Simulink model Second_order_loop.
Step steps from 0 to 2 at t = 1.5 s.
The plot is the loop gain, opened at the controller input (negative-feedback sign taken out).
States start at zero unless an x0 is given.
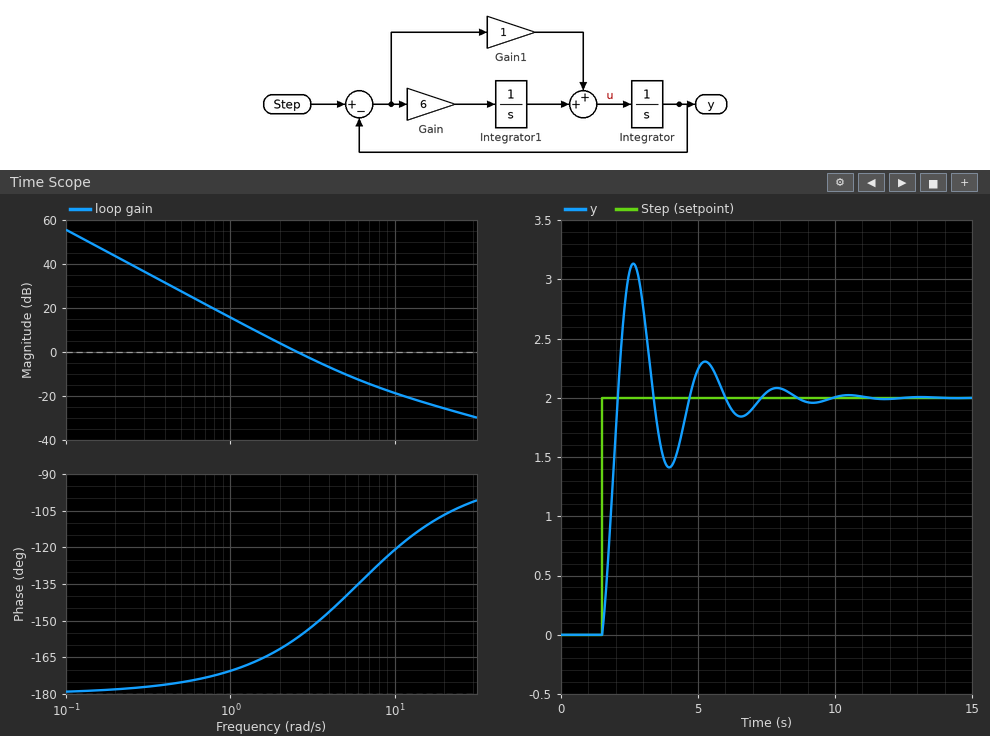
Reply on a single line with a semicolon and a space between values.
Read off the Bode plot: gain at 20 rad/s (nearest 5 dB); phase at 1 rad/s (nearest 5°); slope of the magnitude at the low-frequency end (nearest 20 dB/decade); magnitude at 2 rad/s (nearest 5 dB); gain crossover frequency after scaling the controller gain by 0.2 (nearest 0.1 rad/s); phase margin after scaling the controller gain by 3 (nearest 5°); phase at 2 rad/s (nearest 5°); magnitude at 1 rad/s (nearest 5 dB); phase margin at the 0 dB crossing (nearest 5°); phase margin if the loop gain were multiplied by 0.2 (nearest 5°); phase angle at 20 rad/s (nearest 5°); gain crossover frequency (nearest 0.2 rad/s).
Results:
-25 dB; -170°; -40 dB/decade; 5 dB; 1.1 rad/s; 40°; -160°; 15 dB; 25°; 10°; -105°; 2.6 rad/s
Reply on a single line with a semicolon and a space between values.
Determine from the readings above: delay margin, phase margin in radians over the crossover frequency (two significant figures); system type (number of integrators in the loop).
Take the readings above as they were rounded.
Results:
0.17 s; 2
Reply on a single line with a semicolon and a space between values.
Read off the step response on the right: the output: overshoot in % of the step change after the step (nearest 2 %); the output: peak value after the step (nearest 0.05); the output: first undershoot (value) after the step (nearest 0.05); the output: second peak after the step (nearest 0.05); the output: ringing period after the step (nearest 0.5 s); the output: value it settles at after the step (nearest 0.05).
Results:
56 %; 3.15; 1.40; 2.30; 2.5 s; 2.00
